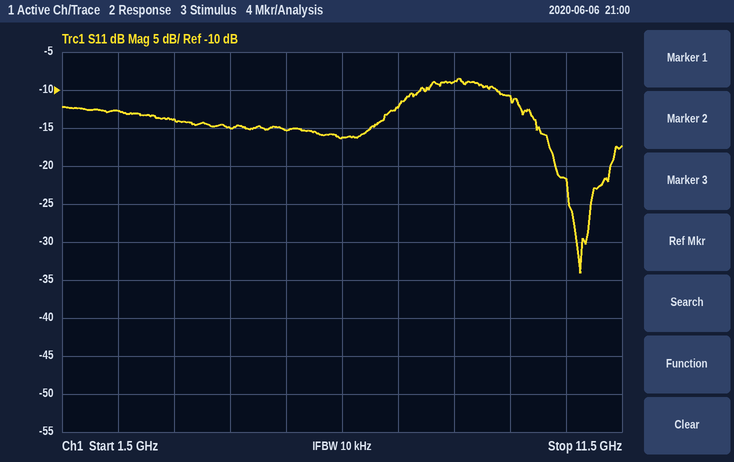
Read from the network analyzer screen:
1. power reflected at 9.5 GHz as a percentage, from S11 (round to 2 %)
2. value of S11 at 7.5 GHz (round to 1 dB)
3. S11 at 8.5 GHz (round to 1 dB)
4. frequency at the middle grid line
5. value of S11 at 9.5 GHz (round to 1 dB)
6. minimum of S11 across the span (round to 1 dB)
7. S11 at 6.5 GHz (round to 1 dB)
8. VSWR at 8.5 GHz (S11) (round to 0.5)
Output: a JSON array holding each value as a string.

["8 %", "-12 dB", "-9 dB", "6.5 GHz", "-11 dB", "-34 dB", "-16 dB", "2.0"]
